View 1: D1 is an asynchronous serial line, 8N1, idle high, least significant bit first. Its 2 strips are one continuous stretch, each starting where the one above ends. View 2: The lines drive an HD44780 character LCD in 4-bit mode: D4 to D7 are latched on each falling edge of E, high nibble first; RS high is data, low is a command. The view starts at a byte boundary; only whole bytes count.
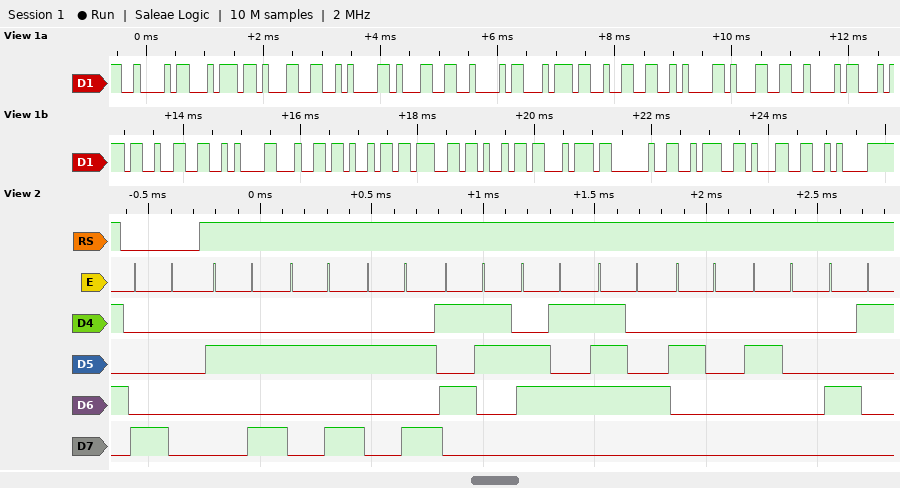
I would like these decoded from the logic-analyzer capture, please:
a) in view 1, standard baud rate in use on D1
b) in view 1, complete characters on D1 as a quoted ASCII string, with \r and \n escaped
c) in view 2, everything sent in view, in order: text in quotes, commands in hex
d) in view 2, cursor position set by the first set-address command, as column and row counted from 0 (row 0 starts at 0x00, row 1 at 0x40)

9600 baud
"Bt1\n1Bt2\n1Bt2\ndigit :1\n"
0x80 "***Set  A"
column 0, row 0
